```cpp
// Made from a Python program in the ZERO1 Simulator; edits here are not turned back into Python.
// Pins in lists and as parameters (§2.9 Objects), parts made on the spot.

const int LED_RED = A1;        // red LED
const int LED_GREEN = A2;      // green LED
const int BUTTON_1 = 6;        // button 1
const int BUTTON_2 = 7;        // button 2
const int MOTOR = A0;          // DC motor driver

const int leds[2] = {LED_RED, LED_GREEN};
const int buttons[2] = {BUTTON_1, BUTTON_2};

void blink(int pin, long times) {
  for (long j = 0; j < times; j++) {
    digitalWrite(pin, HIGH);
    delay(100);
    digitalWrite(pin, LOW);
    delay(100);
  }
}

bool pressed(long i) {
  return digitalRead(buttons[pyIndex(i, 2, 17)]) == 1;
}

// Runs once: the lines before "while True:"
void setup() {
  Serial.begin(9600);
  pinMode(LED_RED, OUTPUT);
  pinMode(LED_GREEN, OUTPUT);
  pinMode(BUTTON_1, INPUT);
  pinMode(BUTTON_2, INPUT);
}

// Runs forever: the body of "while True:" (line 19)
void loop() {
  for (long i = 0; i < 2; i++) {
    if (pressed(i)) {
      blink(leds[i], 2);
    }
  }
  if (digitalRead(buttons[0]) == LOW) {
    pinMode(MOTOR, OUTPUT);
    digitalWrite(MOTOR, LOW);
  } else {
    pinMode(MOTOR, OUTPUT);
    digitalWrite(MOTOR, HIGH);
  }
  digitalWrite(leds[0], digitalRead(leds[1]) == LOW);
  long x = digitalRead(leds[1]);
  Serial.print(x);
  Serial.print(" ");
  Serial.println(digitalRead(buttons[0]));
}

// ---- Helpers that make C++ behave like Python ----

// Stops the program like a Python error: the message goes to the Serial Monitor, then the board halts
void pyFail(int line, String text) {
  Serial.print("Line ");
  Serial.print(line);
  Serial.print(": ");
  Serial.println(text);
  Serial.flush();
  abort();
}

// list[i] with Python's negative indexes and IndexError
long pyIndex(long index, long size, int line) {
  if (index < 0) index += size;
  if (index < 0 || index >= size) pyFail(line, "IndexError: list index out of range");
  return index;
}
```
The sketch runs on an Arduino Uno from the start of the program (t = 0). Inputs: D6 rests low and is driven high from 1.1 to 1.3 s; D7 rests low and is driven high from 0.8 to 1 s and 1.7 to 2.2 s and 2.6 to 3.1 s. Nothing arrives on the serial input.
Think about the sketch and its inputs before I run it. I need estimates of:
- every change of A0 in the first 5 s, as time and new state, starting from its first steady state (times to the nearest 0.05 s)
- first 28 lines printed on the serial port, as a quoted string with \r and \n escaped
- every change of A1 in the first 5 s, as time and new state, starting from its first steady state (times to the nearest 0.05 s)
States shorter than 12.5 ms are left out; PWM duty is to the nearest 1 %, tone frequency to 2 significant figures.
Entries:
0 s low; 1.2 s high; 1.6 s low
"0 0\r\n0 0\r\n0 0\r\n0 0\r\n0 0\r\n0 0\r\n0 0\r\n0 0\r\n0 0\r\n0 0\r\n0 0\r\n0 0\r\n0 0\r\n0 0\r\n0 0\r\n0 0\r\n0 0\r\n0 0\r\n0 0\r\n0 0\r\n0 0\r\n0 0\r\n0 0\r\n0 0\r\n0 0\r\n0 0\r\n0 0\r\n0 0\r\n"
0 s high; 1.3 s low; 1.4 s high; 1.5 s low; 1.6 s high
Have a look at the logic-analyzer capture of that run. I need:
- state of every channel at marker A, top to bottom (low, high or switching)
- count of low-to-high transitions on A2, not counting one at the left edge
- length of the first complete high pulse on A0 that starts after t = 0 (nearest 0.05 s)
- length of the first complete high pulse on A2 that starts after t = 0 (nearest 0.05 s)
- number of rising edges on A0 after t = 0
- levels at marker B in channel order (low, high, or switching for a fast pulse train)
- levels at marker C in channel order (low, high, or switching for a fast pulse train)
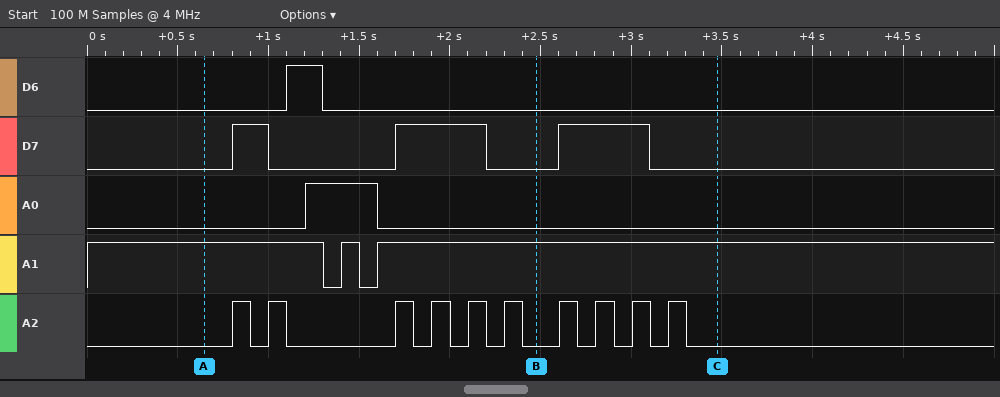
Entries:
D6 low, D7 low, A0 low, A1 high, A2 low
10
0.40 s
0.10 s
1
D6 low, D7 low, A0 low, A1 high, A2 low
D6 low, D7 low, A0 low, A1 high, A2 low
